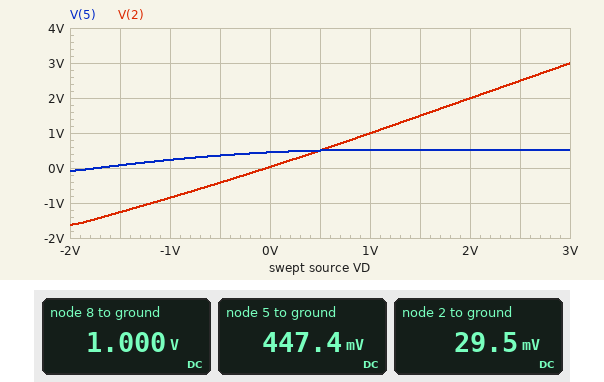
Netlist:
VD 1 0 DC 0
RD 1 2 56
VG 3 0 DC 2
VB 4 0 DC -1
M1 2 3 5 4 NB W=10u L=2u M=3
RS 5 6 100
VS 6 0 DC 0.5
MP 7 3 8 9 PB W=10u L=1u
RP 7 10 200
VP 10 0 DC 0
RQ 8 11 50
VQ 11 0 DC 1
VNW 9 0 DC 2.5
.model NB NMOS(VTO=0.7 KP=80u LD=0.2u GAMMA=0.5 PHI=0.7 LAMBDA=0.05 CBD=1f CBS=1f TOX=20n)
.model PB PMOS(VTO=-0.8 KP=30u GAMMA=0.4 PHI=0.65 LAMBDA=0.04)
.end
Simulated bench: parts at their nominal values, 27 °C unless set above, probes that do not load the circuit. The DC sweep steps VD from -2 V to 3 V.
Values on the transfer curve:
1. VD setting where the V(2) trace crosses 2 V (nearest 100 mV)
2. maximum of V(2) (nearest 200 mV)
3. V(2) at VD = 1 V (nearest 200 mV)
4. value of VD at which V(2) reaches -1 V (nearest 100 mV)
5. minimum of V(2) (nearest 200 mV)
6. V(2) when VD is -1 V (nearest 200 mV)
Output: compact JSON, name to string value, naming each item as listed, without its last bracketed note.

{"VD setting where the V(2) trace crosses 2 V": "2.0 V", "maximum of V(2)": "3.0 V", "V(2) at VD = 1 V": "1.0 V", "value of VD at which V(2) reaches -1 V": "-1.2 V", "minimum of V(2)": "-1.6 V", "V(2) when VD is -1 V": "-800 mV"}
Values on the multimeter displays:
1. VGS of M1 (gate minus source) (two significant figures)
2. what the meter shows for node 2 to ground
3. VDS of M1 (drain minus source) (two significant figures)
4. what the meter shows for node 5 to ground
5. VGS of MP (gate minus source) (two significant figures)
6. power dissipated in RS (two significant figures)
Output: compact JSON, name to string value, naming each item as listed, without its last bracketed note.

{"VGS of M1 (gate minus source)": "1.6 V", "what the meter shows for node 2 to ground": "29.5 mV", "VDS of M1 (drain minus source)": "-420 mV", "what the meter shows for node 5 to ground": "447.4 mV", "VGS of MP (gate minus source)": "1.0 V", "power dissipated in RS": "28 µW"}
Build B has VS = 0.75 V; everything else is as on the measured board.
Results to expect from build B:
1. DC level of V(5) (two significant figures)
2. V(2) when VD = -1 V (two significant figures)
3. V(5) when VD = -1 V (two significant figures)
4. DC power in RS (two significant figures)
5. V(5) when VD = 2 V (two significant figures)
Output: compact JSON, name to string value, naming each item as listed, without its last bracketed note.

{"DC level of V(5)": "680 mV", "V(2) when VD = -1 V": "-830 mV", "V(5) when VD = -1 V": "450 mV", "DC power in RS": "48 µW", "V(5) when VD = 2 V": "750 mV"}
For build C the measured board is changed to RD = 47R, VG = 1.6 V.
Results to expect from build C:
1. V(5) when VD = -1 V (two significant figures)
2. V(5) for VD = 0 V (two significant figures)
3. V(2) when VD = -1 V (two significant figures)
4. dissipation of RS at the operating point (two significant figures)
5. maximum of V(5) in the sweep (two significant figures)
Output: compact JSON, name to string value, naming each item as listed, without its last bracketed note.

{"V(5) when VD = -1 V": "280 mV", "V(5) for VD = 0 V": "470 mV", "V(2) when VD = -1 V": "-900 mV", "dissipation of RS at the operating point": "8.7 µW", "maximum of V(5) in the sweep": "500 mV"}
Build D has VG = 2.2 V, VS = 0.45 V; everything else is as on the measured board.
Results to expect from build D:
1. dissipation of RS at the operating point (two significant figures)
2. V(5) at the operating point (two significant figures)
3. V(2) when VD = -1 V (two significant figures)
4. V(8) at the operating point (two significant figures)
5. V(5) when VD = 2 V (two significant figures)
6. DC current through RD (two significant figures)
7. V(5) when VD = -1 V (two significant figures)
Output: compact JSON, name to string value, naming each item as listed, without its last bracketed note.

{"dissipation of RS at the operating point": "33 µW", "V(5) at the operating point": "390 mV", "V(2) when VD = -1 V": "-840 mV", "V(8) at the operating point": "1.0 V", "V(5) when VD = 2 V": "490 mV", "DC current through RD": "580 µA", "V(5) when VD = -1 V": "170 mV"}
